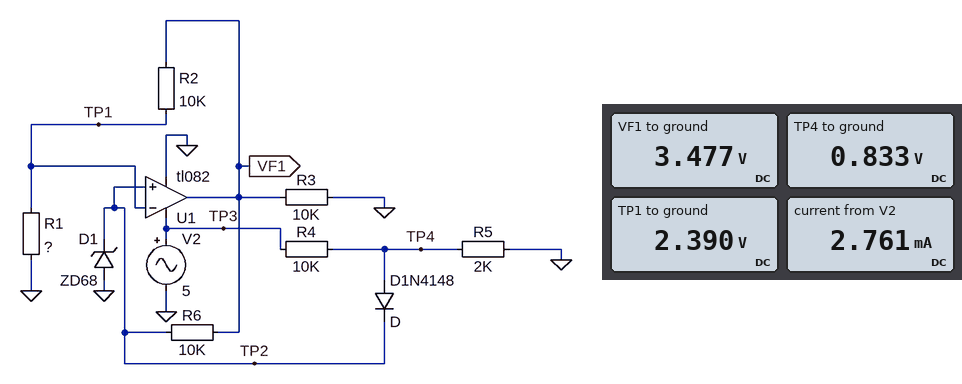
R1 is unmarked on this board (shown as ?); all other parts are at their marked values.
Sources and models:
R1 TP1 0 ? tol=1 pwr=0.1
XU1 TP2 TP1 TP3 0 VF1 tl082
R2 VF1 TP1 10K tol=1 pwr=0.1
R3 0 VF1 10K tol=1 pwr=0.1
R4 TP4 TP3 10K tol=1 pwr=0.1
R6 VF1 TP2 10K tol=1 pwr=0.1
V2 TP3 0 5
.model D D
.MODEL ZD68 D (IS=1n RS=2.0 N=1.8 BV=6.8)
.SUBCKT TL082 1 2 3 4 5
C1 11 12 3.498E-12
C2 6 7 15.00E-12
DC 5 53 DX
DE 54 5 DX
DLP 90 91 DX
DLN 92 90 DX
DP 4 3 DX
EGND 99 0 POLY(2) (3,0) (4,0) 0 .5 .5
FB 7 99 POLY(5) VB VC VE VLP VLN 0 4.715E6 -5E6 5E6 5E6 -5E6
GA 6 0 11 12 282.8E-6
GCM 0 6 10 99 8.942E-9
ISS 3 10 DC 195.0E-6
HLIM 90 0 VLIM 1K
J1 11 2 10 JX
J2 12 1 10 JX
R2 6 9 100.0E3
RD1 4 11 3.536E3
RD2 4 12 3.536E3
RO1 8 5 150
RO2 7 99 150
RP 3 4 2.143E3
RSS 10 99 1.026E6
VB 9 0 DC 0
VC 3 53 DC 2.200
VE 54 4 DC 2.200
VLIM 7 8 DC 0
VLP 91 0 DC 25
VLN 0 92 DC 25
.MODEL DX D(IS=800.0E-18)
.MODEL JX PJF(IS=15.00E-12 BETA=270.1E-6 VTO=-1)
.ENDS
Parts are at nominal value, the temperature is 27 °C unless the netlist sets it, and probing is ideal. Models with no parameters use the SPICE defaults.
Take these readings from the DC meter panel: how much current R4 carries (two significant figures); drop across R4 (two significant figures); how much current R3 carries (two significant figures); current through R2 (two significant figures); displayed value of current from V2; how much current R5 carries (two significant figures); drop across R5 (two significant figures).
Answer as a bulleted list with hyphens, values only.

- 420 µA
- 4.2 V
- 350 µA
- 110 µA
- 2.761 mA
- 420 µA
- 830 mV
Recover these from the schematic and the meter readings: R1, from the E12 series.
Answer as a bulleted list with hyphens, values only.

- 22 kΩ
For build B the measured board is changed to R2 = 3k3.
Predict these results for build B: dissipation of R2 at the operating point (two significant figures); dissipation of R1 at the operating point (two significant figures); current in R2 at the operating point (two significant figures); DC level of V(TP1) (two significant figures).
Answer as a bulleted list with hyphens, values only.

- 62 µW
- 410 µW
- 140 µA
- 3.0 V
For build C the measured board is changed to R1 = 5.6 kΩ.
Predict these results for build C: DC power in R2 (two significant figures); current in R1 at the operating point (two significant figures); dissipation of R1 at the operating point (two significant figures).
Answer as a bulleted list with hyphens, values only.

- 500 µW
- 220 µA
- 280 µW
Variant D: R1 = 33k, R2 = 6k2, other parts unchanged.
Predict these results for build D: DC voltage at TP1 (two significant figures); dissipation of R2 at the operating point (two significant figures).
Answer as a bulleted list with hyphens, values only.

- 2.9 V
- 49 µW
